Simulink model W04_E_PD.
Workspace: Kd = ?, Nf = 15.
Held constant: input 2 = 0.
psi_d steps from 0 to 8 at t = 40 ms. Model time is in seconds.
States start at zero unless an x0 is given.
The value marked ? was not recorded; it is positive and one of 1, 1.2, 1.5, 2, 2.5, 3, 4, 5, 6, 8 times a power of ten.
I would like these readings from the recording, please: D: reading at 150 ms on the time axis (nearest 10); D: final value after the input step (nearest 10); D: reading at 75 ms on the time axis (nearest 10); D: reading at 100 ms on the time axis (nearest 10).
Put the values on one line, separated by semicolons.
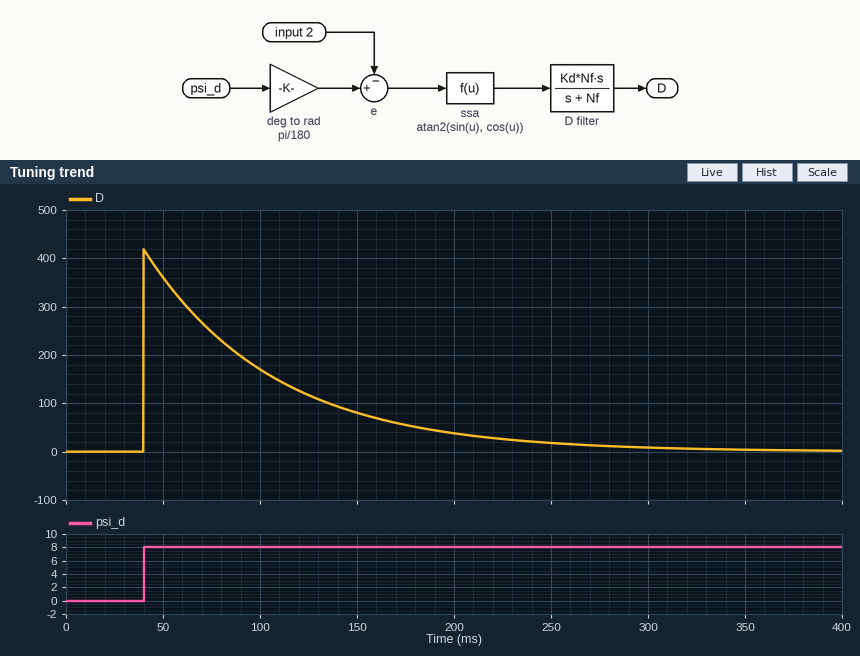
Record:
80; 0; 250; 170
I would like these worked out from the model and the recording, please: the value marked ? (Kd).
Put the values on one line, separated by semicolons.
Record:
200
